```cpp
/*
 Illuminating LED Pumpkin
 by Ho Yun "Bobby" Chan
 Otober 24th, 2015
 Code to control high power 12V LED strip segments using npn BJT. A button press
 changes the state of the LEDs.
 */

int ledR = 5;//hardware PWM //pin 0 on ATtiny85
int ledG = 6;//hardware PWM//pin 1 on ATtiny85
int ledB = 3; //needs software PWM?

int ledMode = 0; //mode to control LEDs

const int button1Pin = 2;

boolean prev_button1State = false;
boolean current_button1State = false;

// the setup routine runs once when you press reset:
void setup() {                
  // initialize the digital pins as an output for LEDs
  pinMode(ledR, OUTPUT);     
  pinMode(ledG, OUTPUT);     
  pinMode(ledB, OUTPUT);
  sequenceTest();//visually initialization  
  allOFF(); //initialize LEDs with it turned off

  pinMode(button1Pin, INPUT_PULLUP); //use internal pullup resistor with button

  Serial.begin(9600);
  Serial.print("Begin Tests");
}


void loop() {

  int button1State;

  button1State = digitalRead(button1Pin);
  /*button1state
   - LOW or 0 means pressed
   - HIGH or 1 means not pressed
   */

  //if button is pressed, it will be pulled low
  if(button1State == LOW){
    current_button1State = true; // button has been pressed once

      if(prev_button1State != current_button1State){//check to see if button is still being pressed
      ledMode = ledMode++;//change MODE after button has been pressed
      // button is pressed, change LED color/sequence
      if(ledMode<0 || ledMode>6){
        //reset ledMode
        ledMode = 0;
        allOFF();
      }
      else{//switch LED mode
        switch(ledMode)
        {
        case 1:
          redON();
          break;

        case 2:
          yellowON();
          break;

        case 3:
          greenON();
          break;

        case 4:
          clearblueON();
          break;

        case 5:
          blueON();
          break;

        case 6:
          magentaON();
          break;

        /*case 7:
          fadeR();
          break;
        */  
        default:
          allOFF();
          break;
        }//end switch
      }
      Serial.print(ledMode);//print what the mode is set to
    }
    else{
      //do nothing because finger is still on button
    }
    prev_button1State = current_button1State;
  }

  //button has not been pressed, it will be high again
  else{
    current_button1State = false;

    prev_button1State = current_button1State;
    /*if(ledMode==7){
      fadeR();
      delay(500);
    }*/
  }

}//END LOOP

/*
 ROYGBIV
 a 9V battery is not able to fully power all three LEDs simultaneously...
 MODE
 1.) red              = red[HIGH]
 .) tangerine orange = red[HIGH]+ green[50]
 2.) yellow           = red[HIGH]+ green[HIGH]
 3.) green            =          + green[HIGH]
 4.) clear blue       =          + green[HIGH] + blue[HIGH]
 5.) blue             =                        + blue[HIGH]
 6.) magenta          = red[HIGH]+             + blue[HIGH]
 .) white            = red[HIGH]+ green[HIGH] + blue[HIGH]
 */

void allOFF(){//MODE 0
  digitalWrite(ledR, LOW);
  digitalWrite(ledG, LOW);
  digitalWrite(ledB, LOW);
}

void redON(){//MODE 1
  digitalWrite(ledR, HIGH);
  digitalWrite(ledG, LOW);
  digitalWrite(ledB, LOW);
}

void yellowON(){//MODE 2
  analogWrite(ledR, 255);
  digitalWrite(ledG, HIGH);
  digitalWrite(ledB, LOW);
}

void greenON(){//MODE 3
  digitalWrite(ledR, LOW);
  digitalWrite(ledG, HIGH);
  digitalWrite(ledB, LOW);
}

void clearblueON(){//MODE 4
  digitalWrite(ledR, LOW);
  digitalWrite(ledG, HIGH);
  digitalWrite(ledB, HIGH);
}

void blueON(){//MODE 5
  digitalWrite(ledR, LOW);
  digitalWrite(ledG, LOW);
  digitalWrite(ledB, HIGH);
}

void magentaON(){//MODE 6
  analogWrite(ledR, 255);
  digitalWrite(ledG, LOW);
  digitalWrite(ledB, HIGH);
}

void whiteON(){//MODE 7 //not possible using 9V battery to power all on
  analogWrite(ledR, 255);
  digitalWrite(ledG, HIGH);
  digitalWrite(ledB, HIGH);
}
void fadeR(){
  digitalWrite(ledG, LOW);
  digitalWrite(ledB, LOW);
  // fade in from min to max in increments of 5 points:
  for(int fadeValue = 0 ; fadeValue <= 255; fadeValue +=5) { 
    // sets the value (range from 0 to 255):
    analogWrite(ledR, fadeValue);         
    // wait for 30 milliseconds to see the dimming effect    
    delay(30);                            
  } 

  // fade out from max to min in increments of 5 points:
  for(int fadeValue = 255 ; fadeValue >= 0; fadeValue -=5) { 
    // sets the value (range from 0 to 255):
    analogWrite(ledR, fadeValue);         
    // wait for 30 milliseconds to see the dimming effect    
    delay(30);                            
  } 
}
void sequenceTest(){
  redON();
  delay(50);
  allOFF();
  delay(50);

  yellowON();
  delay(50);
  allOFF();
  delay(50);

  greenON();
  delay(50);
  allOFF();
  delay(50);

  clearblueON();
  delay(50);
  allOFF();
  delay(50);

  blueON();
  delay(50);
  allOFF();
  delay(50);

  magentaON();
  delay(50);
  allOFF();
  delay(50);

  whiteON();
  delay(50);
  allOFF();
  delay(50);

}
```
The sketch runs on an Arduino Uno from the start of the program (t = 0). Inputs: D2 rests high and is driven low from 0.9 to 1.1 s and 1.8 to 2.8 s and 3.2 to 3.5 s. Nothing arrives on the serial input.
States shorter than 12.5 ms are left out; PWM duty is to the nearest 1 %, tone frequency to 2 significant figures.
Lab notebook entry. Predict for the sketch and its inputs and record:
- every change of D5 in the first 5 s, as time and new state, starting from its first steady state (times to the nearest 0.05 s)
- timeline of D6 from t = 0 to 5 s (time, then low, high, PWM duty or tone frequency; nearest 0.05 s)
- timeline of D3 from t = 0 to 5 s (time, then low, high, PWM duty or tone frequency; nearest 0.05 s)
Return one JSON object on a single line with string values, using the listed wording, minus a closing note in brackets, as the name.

{"every change of D5 in the first 5 s, as time and new state, starting from its first steady state": "0 s high; 0.05 s low; 0.1 s high; 0.15 s low; 0.5 s high; 0.55 s low; 0.6 s high; 0.65 s low", "timeline of D6 from t = 0 to 5 s": "0 s low; 0.1 s high; 0.15 s low; 0.2 s high; 0.25 s low; 0.3 s high; 0.35 s low; 0.6 s high; 0.65 s low", "timeline of D3 from t = 0 to 5 s": "0 s low; 0.3 s high; 0.35 s low; 0.4 s high; 0.45 s low; 0.5 s high; 0.55 s low; 0.6 s high; 0.65 s low"}
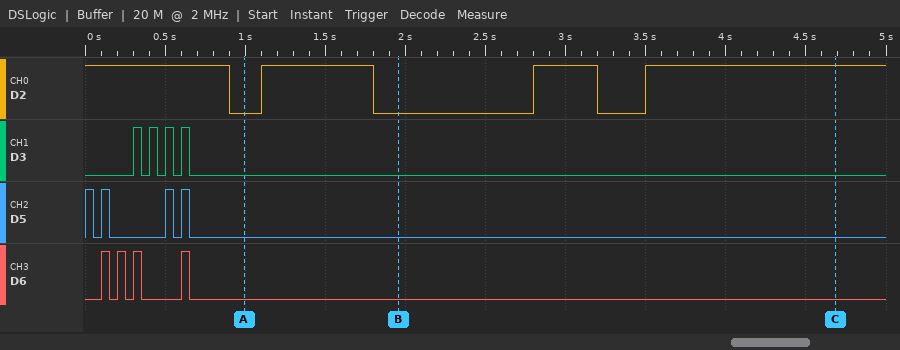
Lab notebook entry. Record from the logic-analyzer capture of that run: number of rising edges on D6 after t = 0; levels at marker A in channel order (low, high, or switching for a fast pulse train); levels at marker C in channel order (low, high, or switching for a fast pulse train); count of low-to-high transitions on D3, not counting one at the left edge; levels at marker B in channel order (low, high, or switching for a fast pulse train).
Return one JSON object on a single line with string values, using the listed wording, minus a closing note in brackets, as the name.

{"number of rising edges on D6 after t = 0": "4", "levels at marker A in channel order": "D2 low, D3 low, D5 low, D6 low", "levels at marker C in channel order": "D2 high, D3 low, D5 low, D6 low", "count of low-to-high transitions on D3, not counting one at the left edge": "4", "levels at marker B in channel order": "D2 low, D3 low, D5 low, D6 low"}
